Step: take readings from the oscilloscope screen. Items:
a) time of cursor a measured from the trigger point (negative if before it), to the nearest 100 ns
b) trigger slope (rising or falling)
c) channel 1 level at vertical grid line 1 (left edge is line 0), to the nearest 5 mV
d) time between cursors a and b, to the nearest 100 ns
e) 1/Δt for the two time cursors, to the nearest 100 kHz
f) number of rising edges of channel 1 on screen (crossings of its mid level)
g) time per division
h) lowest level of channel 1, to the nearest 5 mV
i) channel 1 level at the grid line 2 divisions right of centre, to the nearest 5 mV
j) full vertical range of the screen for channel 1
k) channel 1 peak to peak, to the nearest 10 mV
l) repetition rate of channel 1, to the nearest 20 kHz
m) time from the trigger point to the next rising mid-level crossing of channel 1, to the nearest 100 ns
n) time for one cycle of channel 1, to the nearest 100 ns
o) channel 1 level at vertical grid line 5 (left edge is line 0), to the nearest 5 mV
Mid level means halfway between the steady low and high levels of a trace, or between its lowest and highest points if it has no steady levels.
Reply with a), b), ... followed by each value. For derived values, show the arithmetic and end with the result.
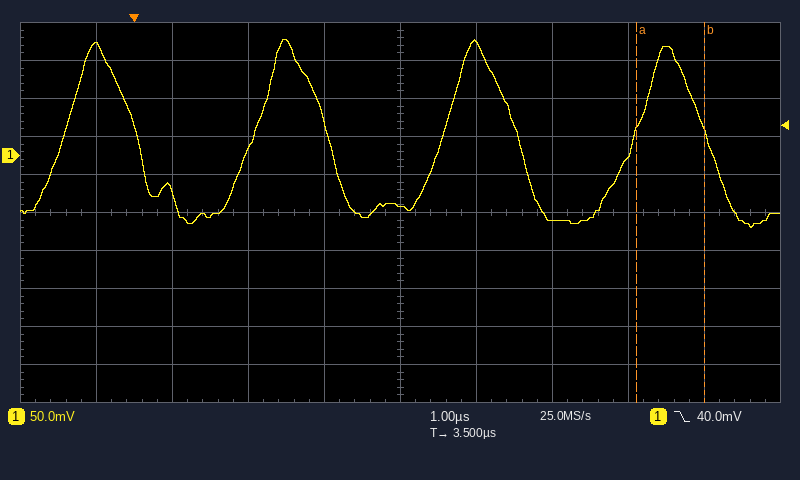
a) +6.6 µs
b) falling
c) 145 mV
d) 900 ns
e) 1 / 900 ns ≈ 1.1 MHz
f) 4
g) 1 µs
h) -95 mV
i) -85 mV
j) 500 mV
k) 250 mV
l) 1 / 2.5 µs ≈ 400 kHz
m) 1.6 µs
n) 2.5 µs
o) -65 mV
